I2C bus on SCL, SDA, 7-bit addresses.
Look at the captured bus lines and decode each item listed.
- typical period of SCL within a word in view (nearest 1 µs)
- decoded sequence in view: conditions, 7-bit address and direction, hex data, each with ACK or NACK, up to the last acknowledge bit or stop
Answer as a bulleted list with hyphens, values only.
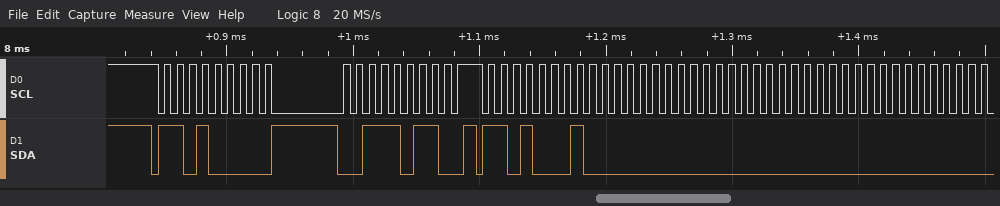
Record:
- 10 µs
- start, address 68 write ACK, 3B ACK, stop, start, address 68 read ACK, 00 ACK, 00 ACK, 00 ACK
